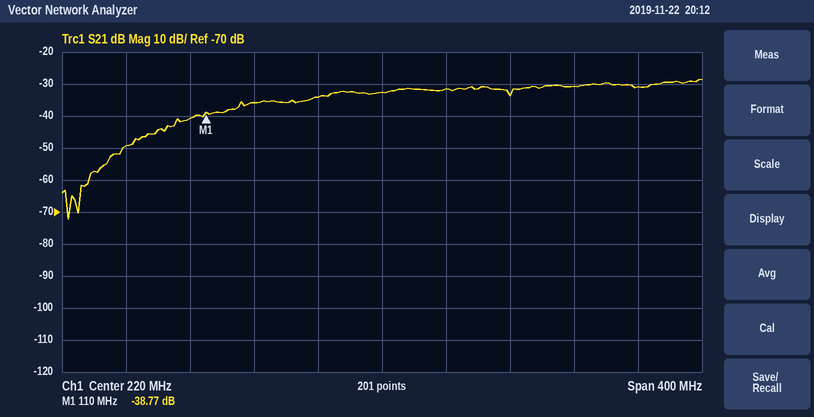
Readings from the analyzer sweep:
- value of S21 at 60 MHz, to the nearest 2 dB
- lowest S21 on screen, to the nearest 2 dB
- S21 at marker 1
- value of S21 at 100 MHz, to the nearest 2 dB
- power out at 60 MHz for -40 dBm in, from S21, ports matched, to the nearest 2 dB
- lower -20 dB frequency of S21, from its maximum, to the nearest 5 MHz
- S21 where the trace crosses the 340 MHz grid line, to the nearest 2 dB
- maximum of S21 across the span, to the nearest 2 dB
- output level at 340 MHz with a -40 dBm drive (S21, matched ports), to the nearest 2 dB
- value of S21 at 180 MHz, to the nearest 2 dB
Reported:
-50 dB
-72 dB
-38.77 dB
-40 dB
-90 dBm
65 MHz
-30 dB
-28 dB
-70 dBm
-34 dB
